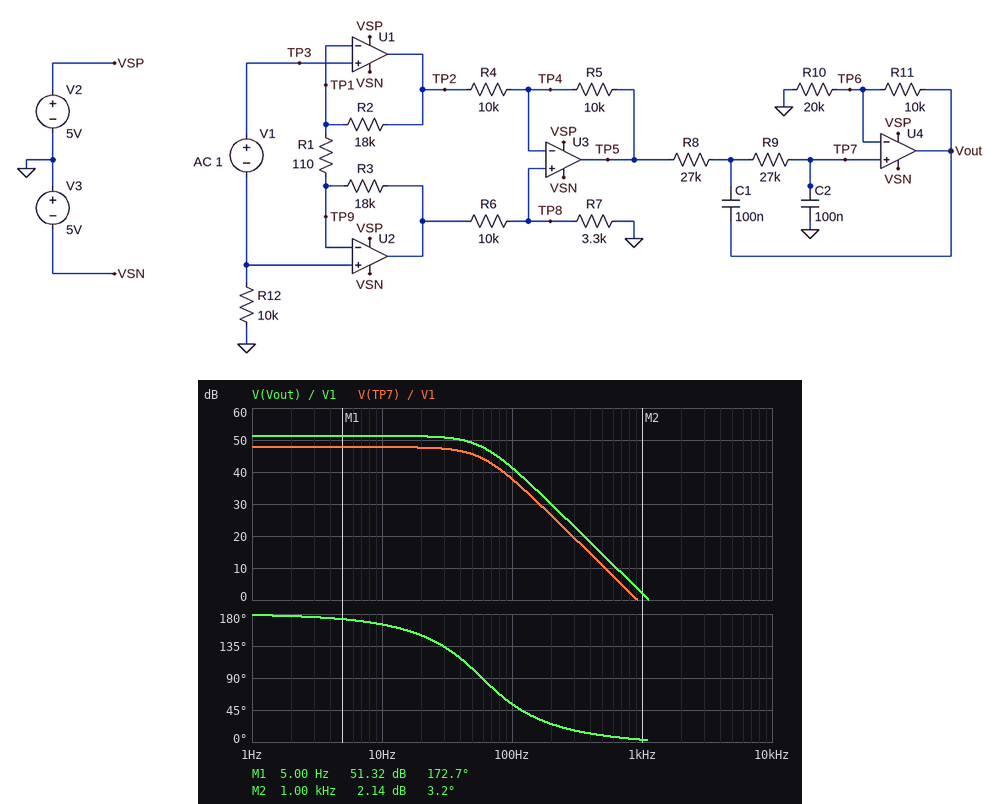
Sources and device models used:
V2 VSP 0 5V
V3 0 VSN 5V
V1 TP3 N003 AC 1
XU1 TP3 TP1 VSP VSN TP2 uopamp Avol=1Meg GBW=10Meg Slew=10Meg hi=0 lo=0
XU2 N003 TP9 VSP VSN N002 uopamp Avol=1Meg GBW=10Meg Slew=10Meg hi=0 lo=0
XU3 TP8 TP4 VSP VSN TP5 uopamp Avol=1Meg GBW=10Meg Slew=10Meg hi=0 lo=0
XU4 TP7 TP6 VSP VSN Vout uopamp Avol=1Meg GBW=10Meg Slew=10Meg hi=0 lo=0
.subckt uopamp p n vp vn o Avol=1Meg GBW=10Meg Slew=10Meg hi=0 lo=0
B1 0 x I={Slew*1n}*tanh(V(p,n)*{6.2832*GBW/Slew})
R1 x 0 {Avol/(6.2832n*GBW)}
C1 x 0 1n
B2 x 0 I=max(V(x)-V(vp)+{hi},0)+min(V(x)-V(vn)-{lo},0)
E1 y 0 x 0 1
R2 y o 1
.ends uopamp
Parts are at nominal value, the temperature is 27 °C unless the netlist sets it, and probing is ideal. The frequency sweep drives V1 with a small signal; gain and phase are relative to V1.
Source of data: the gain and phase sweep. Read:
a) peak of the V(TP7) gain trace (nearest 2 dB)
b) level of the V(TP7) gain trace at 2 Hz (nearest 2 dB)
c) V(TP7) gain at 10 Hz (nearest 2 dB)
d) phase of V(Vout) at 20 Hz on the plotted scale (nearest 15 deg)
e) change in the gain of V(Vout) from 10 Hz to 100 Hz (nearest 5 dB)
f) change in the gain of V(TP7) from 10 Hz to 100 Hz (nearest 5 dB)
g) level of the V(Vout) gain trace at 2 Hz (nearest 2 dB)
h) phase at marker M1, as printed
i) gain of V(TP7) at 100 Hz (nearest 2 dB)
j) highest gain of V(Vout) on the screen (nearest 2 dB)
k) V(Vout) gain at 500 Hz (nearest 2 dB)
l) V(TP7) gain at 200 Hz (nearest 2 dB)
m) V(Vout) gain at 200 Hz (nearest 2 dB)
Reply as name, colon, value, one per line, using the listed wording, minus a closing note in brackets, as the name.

peak of the V(TP7) gain trace: 48 dB
level of the V(TP7) gain trace at 2 Hz: 48 dB
V(TP7) gain at 10 Hz: 48 dB
phase of V(Vout) at 20 Hz on the plotted scale: 150 deg
change in the gain of V(Vout) from 10 Hz to 100 Hz: -10 dB
change in the gain of V(TP7) from 10 Hz to 100 Hz: -10 dB
level of the V(Vout) gain trace at 2 Hz: 52 dB
phase at marker M1, as printed: 172.7 deg
gain of V(TP7) at 100 Hz: 38 dB
highest gain of V(Vout) on the screen: 52 dB
V(Vout) gain at 500 Hz: 14 dB
V(TP7) gain at 200 Hz: 26 dB
V(Vout) gain at 200 Hz: 30 dB
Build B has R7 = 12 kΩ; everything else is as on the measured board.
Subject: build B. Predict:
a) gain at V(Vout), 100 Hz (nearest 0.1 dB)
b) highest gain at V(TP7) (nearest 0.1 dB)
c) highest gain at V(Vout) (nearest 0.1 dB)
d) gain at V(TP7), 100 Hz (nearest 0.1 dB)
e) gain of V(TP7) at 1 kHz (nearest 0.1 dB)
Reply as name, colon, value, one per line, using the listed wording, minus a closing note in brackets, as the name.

gain at V(Vout), 100 Hz: 44.2 dB
highest gain at V(TP7): 50.7 dB
highest gain at V(Vout): 54.2 dB
gain at V(TP7), 100 Hz: 40.7 dB
gain of V(TP7) at 1 kHz: 1.5 dB
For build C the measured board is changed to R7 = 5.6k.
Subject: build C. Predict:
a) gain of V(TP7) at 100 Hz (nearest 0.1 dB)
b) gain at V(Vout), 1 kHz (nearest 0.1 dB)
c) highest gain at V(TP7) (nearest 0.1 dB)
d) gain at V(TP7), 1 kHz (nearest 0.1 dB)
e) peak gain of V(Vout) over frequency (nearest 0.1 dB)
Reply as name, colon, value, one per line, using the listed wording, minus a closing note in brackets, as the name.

gain of V(TP7) at 100 Hz: 39.0 dB
gain at V(Vout), 1 kHz: 3.3 dB
highest gain at V(TP7): 49.0 dB
gain at V(TP7), 1 kHz: -0.2 dB
peak gain of V(Vout) over frequency: 52.5 dB
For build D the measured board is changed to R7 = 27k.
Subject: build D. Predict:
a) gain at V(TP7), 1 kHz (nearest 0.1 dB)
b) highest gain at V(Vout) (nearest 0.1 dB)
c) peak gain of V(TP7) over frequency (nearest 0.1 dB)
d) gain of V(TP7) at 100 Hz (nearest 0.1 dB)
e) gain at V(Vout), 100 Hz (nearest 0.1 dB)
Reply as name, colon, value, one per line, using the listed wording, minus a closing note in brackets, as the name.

gain at V(TP7), 1 kHz: 2.9 dB
highest gain at V(Vout): 55.6 dB
peak gain of V(TP7) over frequency: 52.1 dB
gain of V(TP7) at 100 Hz: 42.1 dB
gain at V(Vout), 100 Hz: 45.6 dB
